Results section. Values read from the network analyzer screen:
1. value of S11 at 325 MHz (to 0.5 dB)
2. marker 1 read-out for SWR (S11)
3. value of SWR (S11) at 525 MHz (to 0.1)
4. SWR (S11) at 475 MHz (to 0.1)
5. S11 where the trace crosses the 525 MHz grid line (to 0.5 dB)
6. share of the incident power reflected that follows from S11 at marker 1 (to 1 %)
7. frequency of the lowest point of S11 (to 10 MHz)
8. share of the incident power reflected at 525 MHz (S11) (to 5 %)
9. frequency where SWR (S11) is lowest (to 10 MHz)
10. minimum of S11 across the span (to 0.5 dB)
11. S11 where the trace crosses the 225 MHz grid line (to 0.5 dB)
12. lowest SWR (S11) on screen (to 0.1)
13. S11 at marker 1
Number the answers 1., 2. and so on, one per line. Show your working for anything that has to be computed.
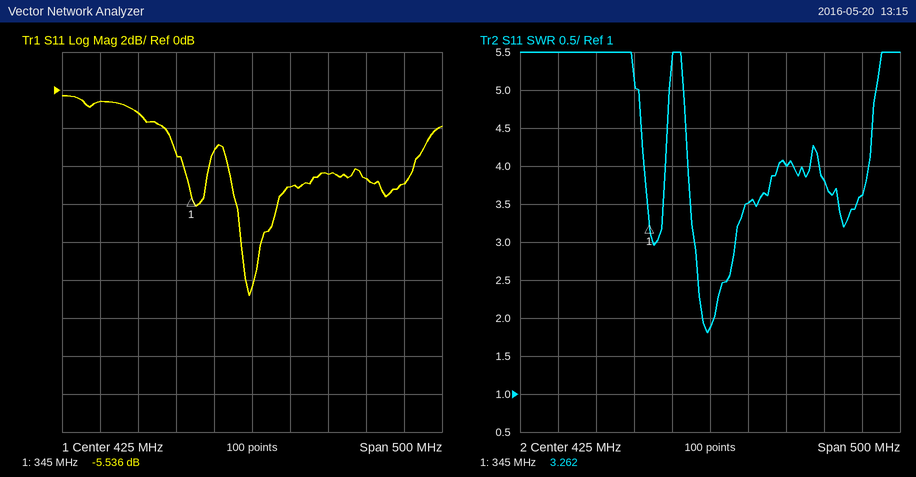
1. -3.5 dB
2. 3.262
3. 4.0
4. 3.5
5. -4.5 dB
6. 10^(-5.536/10) ≈ 28 %
7. 420 MHz
8. 10^(-4.5/10) ≈ 35 %
9. 420 MHz
10. -11.0 dB
11. -0.5 dB
12. 1.8
13. -5.536 dB
